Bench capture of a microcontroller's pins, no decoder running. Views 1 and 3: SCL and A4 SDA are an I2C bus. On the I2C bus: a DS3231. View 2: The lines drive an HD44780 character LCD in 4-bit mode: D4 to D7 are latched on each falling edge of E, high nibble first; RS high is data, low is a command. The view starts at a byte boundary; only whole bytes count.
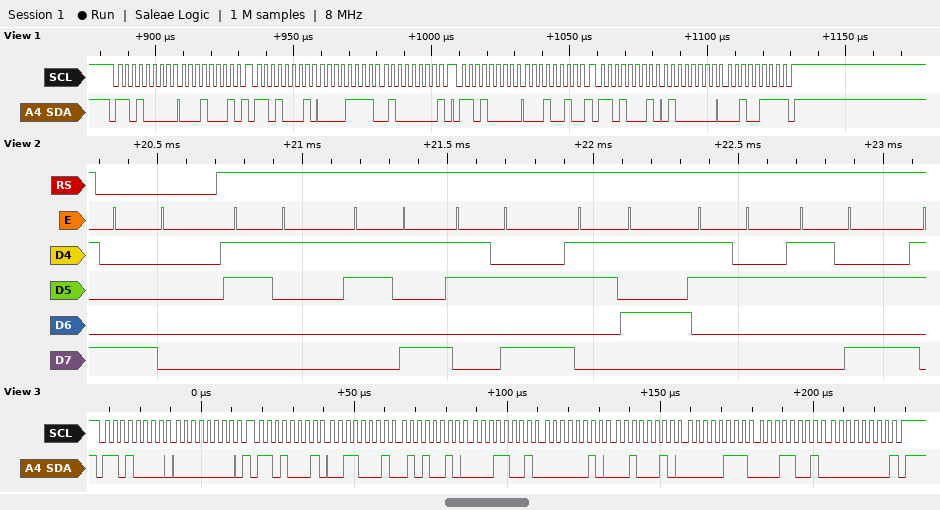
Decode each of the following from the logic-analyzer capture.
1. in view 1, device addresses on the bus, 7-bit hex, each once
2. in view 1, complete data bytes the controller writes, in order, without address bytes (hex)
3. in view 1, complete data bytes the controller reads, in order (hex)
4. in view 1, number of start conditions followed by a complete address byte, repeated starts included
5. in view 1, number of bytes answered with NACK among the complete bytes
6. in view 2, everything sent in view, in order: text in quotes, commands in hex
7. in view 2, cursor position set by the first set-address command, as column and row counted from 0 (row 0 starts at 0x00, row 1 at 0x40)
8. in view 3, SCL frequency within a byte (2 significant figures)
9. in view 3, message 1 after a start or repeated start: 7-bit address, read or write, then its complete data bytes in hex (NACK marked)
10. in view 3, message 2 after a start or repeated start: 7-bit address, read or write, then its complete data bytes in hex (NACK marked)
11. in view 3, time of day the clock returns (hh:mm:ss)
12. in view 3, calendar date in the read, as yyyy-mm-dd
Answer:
0x68
11 12
0F 40 40 27
4
2
0x80 "19:52:"
column 0, row 0
400 kHz
0x68 write: 00
0x68 read: 31 52 19 02 22 07 19 00 NACK
19:52:31
2019-07-22
